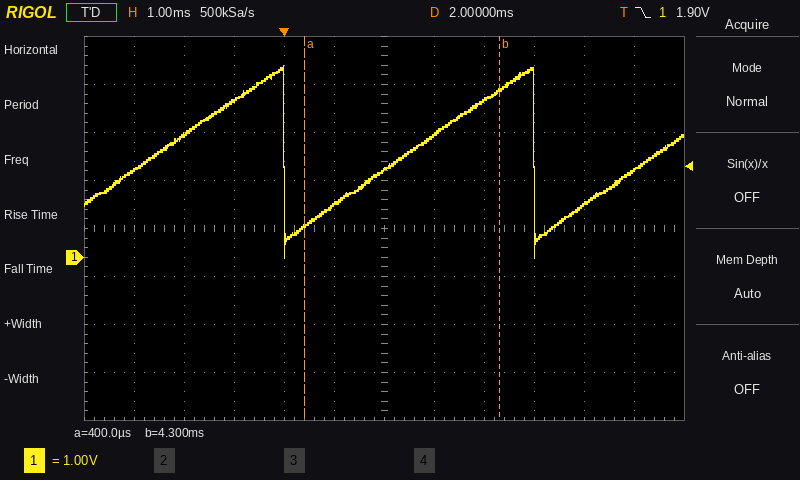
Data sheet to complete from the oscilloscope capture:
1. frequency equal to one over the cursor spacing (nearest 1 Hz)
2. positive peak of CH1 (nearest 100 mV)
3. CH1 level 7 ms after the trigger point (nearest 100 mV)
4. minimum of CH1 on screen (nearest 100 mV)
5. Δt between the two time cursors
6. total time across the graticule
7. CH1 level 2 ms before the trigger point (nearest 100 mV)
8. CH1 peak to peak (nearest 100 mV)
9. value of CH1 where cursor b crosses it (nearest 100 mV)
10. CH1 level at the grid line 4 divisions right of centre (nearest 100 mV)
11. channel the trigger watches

256 Hz
4.0 V
1.8 V
0.0 V
3.9 ms
12 ms
2.6 V
4.0 V
3.5 V
1.1 V
CH1
